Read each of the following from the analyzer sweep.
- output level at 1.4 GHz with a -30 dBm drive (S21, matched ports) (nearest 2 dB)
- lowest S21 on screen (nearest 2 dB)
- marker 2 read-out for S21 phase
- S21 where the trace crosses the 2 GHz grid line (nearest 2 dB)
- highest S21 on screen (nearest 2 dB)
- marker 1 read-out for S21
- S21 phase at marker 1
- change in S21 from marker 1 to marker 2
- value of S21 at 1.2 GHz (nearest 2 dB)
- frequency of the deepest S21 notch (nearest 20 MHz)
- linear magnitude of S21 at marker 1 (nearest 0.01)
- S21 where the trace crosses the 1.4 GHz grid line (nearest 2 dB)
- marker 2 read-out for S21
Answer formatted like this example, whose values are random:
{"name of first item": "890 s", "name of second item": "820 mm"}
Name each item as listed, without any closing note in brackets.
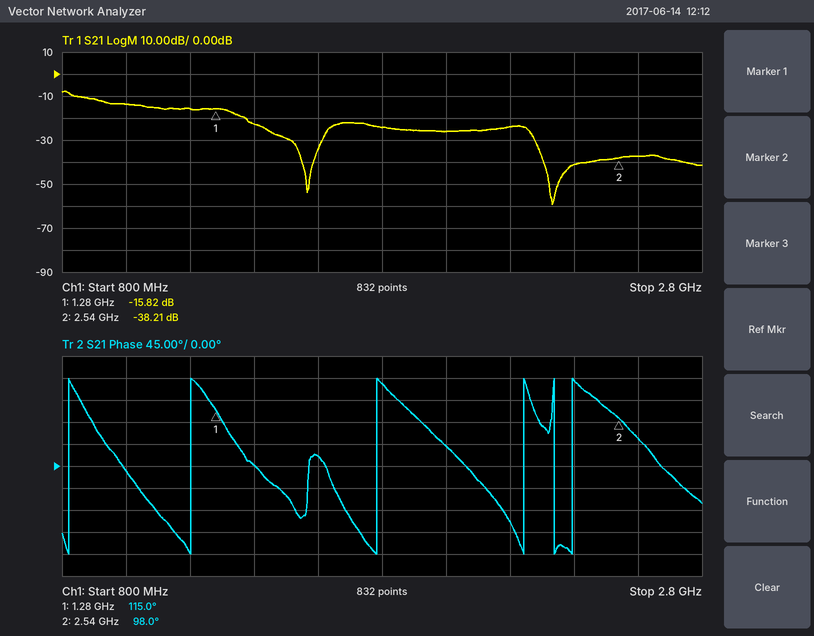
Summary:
{"output level at 1.4 GHz with a -30 dBm drive (S21, matched ports)": "-52 dBm", "lowest S21 on screen": "-60 dB", "marker 2 read-out for S21 phase": "98.0°", "S21 where the trace crosses the 2 GHz grid line": "-26 dB", "highest S21 on screen": "-8 dB", "marker 1 read-out for S21": "-15.82 dB", "S21 phase at marker 1": "115.0°", "change in S21 from marker 1 to marker 2": "-22.39 dB", "value of S21 at 1.2 GHz": "-16 dB", "frequency of the deepest S21 notch": "2.34 GHz", "linear magnitude of S21 at marker 1": "0.16", "S21 where the trace crosses the 1.4 GHz grid line": "-22 dB", "marker 2 read-out for S21": "-38.21 dB"}
